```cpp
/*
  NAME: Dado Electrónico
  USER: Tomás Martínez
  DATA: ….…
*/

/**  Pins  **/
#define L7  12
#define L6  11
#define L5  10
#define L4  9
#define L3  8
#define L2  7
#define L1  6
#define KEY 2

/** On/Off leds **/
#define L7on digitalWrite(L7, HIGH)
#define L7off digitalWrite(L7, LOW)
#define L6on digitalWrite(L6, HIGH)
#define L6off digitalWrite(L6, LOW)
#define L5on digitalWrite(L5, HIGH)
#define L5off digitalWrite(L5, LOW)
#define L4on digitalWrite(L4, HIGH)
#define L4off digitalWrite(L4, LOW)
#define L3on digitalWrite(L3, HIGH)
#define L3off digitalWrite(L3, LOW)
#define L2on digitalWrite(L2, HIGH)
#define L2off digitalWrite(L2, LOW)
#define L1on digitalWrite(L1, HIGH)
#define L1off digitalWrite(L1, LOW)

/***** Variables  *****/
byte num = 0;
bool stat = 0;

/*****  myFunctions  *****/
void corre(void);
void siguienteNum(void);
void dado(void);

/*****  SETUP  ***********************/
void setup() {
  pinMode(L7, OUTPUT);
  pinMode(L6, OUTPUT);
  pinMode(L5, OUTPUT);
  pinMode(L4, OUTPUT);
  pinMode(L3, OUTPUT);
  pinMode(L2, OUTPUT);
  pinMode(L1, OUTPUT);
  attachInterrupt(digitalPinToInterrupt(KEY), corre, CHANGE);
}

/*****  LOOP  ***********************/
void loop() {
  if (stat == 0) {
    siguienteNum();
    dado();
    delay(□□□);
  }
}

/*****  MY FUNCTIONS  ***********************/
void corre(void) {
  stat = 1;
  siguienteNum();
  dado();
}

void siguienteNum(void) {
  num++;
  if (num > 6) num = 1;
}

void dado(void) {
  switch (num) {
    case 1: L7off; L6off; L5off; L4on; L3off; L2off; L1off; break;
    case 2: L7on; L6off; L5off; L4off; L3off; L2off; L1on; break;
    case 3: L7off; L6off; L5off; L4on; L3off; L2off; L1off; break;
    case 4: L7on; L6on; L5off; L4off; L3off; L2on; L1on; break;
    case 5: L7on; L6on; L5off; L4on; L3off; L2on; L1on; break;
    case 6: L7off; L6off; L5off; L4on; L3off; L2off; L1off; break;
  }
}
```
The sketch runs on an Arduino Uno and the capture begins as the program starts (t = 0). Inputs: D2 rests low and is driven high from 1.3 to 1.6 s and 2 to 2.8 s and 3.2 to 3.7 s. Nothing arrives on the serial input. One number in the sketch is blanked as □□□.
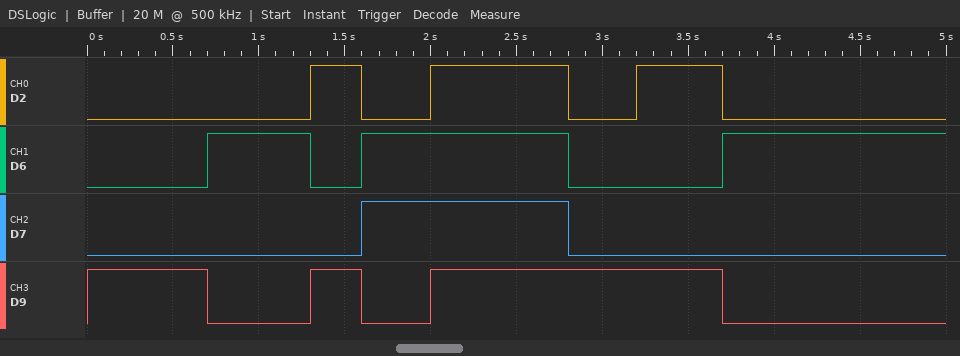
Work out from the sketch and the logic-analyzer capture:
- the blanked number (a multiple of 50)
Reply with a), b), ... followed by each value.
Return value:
a) 700
